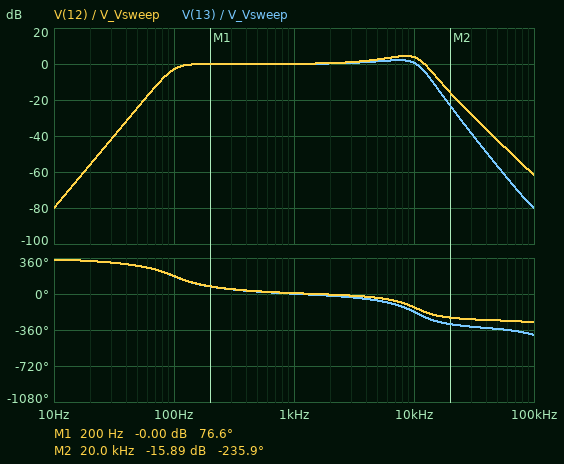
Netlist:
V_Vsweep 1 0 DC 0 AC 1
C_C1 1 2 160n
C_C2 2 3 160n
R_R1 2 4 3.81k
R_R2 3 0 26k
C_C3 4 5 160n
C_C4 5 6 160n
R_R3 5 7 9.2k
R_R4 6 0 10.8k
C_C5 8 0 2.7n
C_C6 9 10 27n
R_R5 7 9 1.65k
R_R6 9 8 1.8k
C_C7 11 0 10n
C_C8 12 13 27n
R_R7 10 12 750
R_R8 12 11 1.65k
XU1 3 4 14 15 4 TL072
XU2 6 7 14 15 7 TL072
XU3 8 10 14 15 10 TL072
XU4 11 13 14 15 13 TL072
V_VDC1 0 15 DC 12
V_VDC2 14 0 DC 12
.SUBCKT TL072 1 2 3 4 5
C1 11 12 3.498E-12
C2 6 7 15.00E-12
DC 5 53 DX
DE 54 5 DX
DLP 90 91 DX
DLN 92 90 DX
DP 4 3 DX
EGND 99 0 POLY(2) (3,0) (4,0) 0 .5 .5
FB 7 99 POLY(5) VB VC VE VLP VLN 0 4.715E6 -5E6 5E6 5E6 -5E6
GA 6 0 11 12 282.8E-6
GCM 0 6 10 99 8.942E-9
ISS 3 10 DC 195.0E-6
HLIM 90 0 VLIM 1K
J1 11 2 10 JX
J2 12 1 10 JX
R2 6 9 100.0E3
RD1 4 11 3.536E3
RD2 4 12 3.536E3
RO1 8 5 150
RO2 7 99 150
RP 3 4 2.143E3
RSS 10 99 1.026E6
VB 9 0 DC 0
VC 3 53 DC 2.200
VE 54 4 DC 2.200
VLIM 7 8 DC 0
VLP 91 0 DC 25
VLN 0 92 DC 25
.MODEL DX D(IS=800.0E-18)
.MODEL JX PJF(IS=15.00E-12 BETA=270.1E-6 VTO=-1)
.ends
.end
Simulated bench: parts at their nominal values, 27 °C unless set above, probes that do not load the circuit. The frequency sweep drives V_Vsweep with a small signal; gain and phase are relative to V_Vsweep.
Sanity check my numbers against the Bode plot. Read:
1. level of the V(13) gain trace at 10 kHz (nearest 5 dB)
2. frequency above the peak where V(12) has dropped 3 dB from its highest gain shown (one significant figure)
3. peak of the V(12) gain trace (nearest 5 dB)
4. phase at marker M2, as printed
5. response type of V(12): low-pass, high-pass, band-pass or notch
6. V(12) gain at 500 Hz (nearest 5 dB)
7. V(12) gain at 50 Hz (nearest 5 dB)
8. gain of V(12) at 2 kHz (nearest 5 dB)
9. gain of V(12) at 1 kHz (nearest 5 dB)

0 dB
10 kHz
5 dB
-235.9 deg
band-pass
0 dB
-25 dB
0 dB
0 dB
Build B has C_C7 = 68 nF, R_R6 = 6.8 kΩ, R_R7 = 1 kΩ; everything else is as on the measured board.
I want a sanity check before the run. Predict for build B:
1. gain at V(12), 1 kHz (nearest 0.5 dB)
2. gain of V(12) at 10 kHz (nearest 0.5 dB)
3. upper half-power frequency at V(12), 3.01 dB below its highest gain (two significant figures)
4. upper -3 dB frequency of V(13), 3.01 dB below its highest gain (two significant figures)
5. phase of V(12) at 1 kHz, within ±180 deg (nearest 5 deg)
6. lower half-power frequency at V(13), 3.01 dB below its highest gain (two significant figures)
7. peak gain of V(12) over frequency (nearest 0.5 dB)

-1.0 dB
-15.5 dB
5.8 kHz
1.1 kHz
-10 deg
99 Hz
0 dB
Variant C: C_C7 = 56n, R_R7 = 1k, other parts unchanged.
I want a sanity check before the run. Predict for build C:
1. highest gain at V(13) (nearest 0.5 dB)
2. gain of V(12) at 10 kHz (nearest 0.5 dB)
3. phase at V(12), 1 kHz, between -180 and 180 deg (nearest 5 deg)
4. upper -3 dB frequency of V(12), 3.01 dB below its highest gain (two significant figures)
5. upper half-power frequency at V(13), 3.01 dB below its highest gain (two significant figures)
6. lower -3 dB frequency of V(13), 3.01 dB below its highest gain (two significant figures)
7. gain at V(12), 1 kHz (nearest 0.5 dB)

0 dB
-2.5 dB
-5 deg
11 kHz
1.3 kHz
99 Hz
-1.0 dB
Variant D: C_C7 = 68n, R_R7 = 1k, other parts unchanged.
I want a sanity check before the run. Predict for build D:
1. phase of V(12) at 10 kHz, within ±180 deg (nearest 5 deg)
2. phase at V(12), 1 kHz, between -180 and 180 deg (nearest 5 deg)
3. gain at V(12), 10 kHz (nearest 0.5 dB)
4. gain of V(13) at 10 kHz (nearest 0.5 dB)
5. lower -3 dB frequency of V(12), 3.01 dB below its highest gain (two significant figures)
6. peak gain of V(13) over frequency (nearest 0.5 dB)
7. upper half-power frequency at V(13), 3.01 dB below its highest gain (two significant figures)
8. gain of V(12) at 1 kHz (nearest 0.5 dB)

-130 deg
-5 deg
-2.5 dB
-19.5 dB
99 Hz
0 dB
1.0 kHz
-1.5 dB
